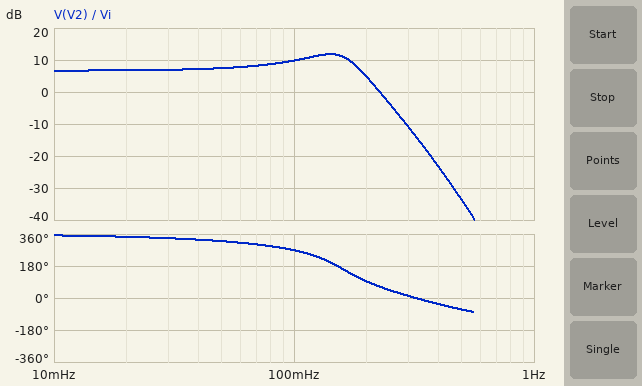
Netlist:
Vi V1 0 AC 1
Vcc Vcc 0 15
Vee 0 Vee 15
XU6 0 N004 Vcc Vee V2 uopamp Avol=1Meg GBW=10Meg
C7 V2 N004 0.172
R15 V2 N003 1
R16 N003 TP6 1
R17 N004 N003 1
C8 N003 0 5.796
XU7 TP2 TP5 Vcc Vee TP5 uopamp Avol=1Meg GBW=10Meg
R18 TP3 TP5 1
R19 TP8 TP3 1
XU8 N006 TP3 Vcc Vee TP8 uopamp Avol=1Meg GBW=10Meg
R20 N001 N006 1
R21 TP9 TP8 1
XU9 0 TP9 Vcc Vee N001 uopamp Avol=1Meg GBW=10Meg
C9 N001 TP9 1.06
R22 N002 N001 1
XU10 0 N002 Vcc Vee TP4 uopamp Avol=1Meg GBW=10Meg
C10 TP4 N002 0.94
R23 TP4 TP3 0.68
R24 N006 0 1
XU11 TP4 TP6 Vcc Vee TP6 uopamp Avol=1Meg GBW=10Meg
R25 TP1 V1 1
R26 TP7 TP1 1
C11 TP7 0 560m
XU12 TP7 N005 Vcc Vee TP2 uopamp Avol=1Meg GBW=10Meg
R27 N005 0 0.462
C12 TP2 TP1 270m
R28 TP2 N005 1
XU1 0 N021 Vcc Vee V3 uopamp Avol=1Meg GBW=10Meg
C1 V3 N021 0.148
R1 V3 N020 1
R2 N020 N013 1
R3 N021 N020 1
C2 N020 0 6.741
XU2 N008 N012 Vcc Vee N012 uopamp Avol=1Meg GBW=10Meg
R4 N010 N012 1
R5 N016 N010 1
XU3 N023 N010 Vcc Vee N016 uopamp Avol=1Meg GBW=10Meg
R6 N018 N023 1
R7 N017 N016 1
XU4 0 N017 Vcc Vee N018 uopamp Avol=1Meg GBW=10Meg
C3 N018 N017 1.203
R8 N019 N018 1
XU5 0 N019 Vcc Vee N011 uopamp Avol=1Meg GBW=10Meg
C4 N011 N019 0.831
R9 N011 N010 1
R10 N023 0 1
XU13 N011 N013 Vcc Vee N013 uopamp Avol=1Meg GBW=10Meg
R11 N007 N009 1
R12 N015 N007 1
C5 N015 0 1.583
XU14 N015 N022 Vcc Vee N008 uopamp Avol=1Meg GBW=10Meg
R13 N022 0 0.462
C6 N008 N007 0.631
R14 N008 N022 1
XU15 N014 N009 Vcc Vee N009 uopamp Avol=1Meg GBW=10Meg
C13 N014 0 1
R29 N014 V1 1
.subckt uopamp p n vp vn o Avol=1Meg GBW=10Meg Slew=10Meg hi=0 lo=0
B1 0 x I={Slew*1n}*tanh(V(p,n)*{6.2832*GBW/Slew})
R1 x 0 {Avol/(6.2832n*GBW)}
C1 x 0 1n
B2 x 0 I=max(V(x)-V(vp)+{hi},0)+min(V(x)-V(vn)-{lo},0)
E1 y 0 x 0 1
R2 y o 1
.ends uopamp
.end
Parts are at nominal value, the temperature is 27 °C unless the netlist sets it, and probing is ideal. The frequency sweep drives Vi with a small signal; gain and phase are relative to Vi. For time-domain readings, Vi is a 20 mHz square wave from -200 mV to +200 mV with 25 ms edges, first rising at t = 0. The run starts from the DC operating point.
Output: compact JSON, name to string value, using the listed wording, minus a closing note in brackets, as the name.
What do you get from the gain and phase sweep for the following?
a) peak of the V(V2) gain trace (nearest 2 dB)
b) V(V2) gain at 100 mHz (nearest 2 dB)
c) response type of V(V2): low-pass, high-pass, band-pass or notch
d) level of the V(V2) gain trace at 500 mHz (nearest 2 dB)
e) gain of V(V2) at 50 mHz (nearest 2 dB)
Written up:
{"peak of the V(V2) gain trace": "12 dB", "V(V2) gain at 100 mHz": "10 dB", "response type of V(V2): low-pass, high-pass, band-pass or notch": "low-pass", "level of the V(V2) gain trace at 500 mHz": "-34 dB", "gain of V(V2) at 50 mHz": "8 dB"}
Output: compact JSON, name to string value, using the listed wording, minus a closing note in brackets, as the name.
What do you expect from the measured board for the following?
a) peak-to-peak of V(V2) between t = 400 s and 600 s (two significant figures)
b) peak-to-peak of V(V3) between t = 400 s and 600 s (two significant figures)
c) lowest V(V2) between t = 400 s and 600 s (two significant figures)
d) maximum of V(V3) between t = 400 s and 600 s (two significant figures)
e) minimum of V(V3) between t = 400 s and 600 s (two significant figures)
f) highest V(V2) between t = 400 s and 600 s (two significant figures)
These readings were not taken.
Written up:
{"peak-to-peak of V(V2) between t = 400 s and 600 s": "1.6 V", "peak-to-peak of V(V3) between t = 400 s and 600 s": "1.7 V", "lowest V(V2) between t = 400 s and 600 s": "-780 mV", "maximum of V(V3) between t = 400 s and 600 s": "830 mV", "minimum of V(V3) between t = 400 s and 600 s": "-830 mV", "highest V(V2) between t = 400 s and 600 s": "780 mV"}
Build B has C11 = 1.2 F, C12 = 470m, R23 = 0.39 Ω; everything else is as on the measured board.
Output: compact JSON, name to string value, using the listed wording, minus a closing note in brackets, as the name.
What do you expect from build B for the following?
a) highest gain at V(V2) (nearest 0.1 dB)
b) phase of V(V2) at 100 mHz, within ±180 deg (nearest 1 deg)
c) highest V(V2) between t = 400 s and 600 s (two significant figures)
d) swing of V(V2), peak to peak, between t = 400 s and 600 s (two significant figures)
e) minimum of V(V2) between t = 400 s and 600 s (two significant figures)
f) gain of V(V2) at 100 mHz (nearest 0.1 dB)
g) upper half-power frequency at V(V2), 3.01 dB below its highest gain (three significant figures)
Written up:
{"highest gain at V(V2)": "5.0 dB", "phase of V(V2) at 100 mHz, within ±180 deg": "-108 deg", "highest V(V2) between t = 400 s and 600 s": "390 mV", "swing of V(V2), peak to peak, between t = 400 s and 600 s": "780 mV", "minimum of V(V2) between t = 400 s and 600 s": "-390 mV", "gain of V(V2) at 100 mHz": "3.8 dB", "upper half-power frequency at V(V2), 3.01 dB below its highest gain": "174 mHz"}
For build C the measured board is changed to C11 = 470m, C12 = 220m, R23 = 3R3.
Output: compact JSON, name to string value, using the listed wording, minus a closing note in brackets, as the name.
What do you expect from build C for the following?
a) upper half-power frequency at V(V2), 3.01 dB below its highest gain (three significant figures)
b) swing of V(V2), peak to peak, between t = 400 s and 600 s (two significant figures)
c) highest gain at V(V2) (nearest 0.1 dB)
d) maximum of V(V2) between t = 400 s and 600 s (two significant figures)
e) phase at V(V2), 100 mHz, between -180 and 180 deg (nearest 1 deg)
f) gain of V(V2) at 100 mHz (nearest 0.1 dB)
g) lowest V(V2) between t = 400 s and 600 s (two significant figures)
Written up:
{"upper half-power frequency at V(V2), 3.01 dB below its highest gain": "77.9 mHz", "swing of V(V2), peak to peak, between t = 400 s and 600 s": "4.2 V", "highest gain at V(V2)": "20.4 dB", "maximum of V(V2) between t = 400 s and 600 s": "2.1 V", "phase at V(V2), 100 mHz, between -180 and 180 deg": "-143 deg", "gain of V(V2) at 100 mHz": "16.5 dB", "lowest V(V2) between t = 400 s and 600 s": "-2.1 V"}
